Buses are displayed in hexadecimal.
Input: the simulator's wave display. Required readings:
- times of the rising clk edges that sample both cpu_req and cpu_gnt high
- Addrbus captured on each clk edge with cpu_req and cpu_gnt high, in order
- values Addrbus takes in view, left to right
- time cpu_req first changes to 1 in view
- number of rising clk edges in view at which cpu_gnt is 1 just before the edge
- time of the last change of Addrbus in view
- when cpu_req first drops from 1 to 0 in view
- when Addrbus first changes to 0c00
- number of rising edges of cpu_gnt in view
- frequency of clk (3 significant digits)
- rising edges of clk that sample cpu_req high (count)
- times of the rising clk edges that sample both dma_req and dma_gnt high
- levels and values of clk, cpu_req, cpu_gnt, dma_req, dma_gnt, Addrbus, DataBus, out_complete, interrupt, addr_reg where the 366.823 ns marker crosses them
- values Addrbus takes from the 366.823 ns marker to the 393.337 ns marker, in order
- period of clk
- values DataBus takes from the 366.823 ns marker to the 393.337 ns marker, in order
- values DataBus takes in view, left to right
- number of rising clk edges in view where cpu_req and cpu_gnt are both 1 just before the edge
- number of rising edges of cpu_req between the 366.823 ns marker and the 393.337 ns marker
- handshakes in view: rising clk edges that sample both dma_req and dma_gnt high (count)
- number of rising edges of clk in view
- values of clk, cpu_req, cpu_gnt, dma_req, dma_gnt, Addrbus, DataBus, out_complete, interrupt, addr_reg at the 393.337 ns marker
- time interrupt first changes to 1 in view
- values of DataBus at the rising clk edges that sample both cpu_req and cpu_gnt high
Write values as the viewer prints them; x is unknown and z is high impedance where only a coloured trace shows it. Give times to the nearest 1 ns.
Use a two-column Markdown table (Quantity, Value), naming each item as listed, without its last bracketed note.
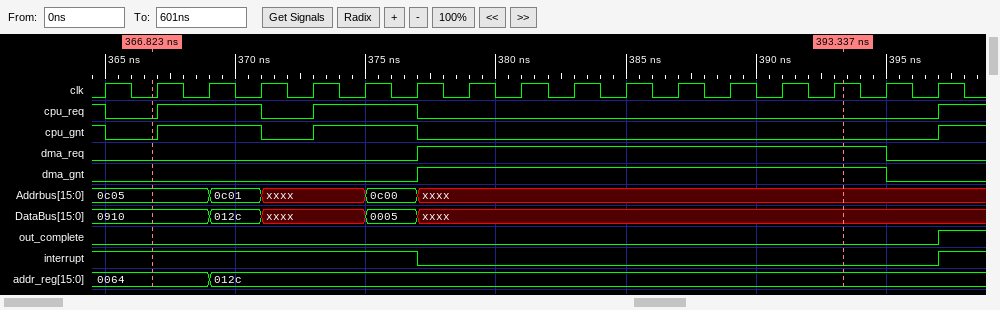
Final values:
| Quantity | Value |
|---|---|
| times of the rising clk edges that sample both cpu_req and cpu_gnt high | 365 ns, 369 ns, 371 ns, 375 ns, 377 ns |
| Addrbus captured on each clk edge with cpu_req and cpu_gnt high, in order | 0c05, 0c05, 0c01, xxxx, 0c00 |
| values Addrbus takes in view, left to right | 0c05, 0c01, xxxx, 0c00, xxxx |
| time cpu_req first changes to 1 in view | 367 ns |
| number of rising clk edges in view at which cpu_gnt is 1 just before the edge | 5 |
| time of the last change of Addrbus in view | 377 ns |
| when cpu_req first drops from 1 to 0 in view | 365 ns |
| when Addrbus first changes to 0c00 | 375 ns |
| number of rising edges of cpu_gnt in view | 3 |
| frequency of clk | 500 MHz |
| rising edges of clk that sample cpu_req high | 5 |
| times of the rising clk edges that sample both dma_req and dma_gnt high | 379 ns, 381 ns, 383 ns, 385 ns, 387 ns, 389 ns, 391 ns, 393 ns, 395 ns |
| levels and values of clk, cpu_req, cpu_gnt, dma_req, dma_gnt, Addrbus, DataBus, out_complete, interrupt, addr_reg where the 366.823 ns marker crosses them | clk=0, cpu_req=0, cpu_gnt=0, dma_req=0, dma_gnt=0, Addrbus=0c05, DataBus=0910, out_complete=0, interrupt=1, addr_reg=0064 |
| values Addrbus takes from the 366.823 ns marker to the 393.337 ns marker, in order | 0c05, 0c01, xxxx, 0c00, xxxx |
| period of clk | 2 ns |
| values DataBus takes from the 366.823 ns marker to the 393.337 ns marker, in order | 0910, 012c, xxxx, 0005, xxxx |
| values DataBus takes in view, left to right | 0910, 012c, xxxx, 0005, xxxx |
| number of rising clk edges in view where cpu_req and cpu_gnt are both 1 just before the edge | 5 |
| number of rising edges of cpu_req between the 366.823 ns marker and the 393.337 ns marker | 2 |
| handshakes in view: rising clk edges that sample both dma_req and dma_gnt high | 9 |
| number of rising edges of clk in view | 17 |
| values of clk, cpu_req, cpu_gnt, dma_req, dma_gnt, Addrbus, DataBus, out_complete, interrupt, addr_reg at the 393.337 ns marker | clk=1, cpu_req=0, cpu_gnt=0, dma_req=1, dma_gnt=1, Addrbus=xxxx, DataBus=xxxx, out_complete=0, interrupt=0, addr_reg=012c |
| time interrupt first changes to 1 in view | 397 ns |
| values of DataBus at the rising clk edges that sample both cpu_req and cpu_gnt high | 0910, 0910, 012c, xxxx, 0005 |
